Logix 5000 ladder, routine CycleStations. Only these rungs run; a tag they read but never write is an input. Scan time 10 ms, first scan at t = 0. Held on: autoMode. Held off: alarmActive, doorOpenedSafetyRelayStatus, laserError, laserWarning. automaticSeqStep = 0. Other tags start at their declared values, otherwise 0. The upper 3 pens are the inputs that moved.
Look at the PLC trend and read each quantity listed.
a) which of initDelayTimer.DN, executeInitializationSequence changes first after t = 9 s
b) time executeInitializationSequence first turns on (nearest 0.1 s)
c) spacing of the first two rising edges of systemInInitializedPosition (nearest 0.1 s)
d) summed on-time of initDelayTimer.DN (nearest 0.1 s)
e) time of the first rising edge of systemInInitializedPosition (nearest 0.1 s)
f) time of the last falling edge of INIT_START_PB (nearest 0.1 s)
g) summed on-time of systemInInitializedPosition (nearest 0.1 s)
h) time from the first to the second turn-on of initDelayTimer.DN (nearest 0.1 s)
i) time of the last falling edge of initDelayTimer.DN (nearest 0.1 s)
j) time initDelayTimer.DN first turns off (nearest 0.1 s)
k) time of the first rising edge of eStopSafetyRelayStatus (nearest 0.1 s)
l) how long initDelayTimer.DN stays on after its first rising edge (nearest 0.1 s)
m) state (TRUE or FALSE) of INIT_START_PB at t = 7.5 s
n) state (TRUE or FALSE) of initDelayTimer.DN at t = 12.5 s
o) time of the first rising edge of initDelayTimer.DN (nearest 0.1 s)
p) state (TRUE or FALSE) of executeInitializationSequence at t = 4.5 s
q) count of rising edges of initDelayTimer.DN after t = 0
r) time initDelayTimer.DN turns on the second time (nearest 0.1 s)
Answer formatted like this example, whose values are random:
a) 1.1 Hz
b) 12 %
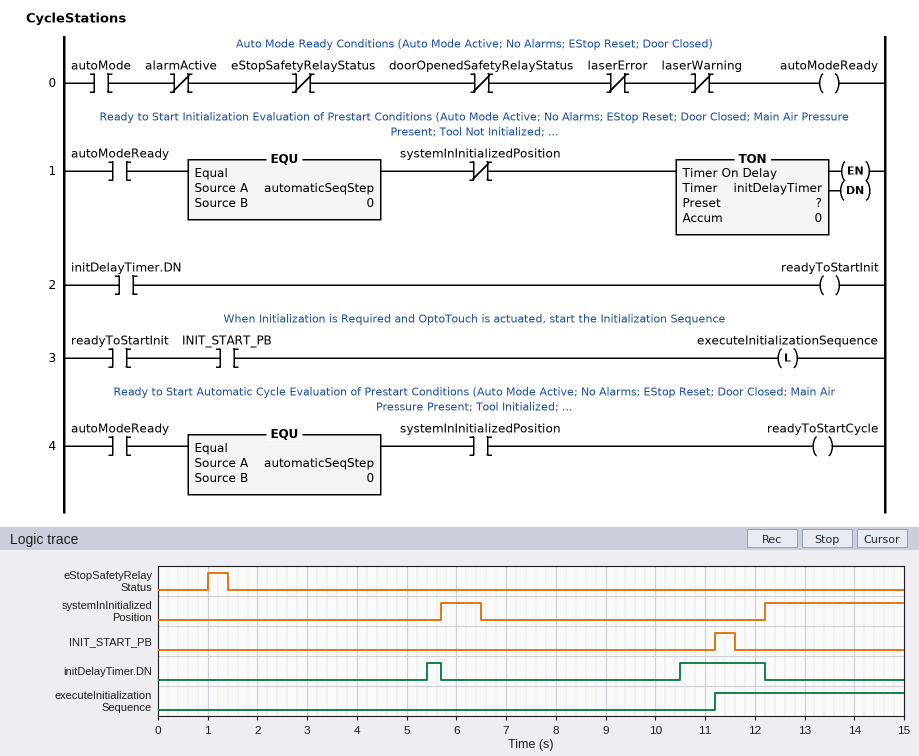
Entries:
a) initDelayTimer.DN
b) 11.2 s
c) 6.5 s
d) 2.0 s
e) 5.7 s
f) 11.6 s
g) 3.6 s
h) 5.1 s
i) 12.2 s
j) 5.7 s
k) 1.0 s
l) 0.3 s
m) FALSE
n) FALSE
o) 5.4 s
p) FALSE
q) 2
r) 10.5 s
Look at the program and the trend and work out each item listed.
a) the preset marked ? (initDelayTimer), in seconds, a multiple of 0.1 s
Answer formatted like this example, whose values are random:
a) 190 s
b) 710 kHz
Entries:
a) 4.0 s
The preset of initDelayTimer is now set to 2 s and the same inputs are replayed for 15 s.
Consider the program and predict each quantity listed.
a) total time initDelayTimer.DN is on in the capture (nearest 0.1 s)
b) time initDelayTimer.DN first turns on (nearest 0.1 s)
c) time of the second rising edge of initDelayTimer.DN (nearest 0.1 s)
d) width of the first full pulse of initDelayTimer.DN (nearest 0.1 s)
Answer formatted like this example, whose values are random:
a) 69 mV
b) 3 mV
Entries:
a) 6.0 s
b) 3.4 s
c) 8.5 s
d) 2.3 s
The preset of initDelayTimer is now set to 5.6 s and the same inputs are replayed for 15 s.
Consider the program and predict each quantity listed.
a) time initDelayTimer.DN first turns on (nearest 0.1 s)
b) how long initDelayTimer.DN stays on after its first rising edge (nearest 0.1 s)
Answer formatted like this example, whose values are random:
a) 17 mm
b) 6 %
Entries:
a) 12.1 s
b) 0.1 s
